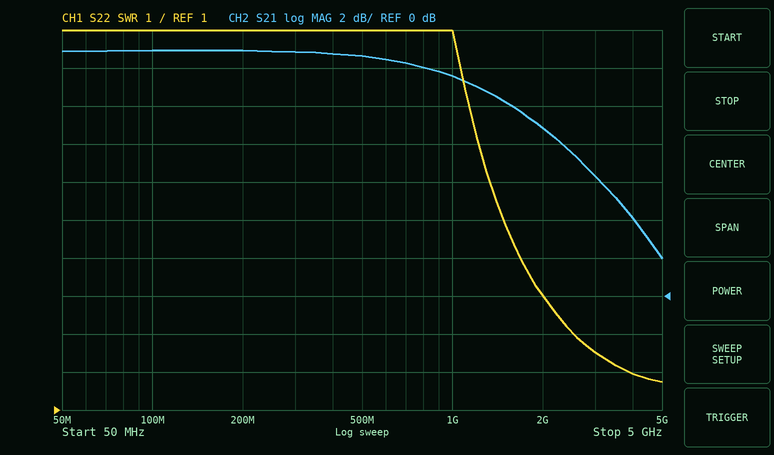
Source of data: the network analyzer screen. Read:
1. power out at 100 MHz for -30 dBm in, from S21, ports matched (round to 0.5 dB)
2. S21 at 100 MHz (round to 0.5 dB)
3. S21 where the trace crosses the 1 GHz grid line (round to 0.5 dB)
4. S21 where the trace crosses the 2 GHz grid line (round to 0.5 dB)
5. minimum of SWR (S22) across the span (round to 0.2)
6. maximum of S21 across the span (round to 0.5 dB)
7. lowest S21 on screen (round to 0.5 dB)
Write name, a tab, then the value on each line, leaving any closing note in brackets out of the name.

power out at 100 MHz for -30 dBm in, from S21, ports matched	-17.0 dBm
S21 at 100 MHz	13.0 dB
S21 where the trace crosses the 1 GHz grid line	11.5 dB
S21 where the trace crosses the 2 GHz grid line	9.0 dB
minimum of SWR (S22) across the span	1.8
maximum of S21 across the span	13.0 dB
lowest S21 on screen	2.0 dB
